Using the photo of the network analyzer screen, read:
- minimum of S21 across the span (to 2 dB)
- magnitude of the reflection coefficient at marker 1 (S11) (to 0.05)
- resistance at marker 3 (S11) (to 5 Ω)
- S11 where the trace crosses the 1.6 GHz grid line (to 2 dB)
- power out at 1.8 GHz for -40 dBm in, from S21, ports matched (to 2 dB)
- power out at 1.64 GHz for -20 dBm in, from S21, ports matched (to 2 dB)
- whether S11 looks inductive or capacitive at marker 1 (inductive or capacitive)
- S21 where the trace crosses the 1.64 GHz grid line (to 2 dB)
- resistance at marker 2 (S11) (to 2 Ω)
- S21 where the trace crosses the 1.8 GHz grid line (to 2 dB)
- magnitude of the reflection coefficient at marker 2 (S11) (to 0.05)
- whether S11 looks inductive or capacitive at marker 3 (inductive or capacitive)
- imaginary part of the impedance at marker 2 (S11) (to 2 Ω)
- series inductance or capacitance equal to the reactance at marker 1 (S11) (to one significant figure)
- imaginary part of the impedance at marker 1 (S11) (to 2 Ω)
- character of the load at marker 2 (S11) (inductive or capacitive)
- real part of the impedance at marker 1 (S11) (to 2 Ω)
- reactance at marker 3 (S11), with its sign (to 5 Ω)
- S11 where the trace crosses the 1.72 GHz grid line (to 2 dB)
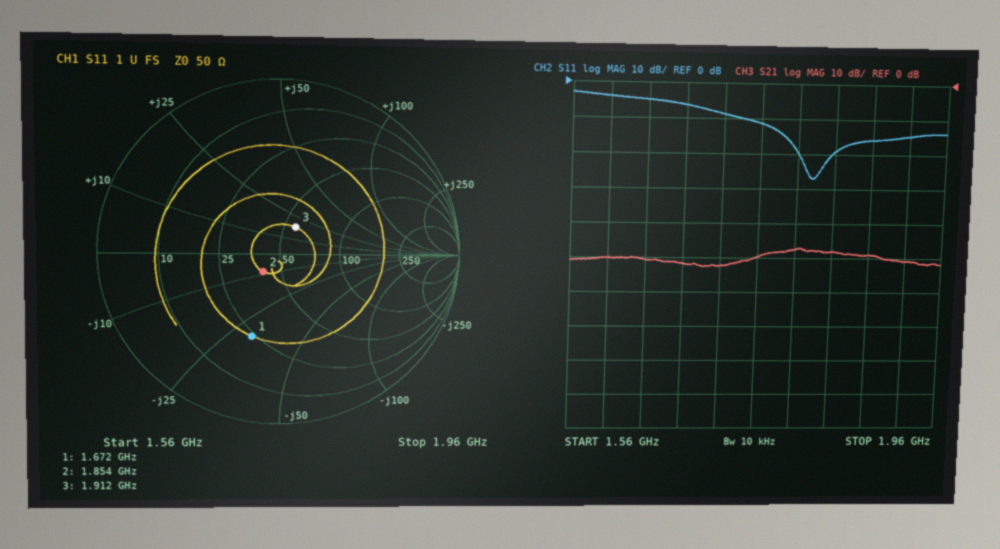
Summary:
-52 dB
0.50
55 Ω
-4 dB
-88 dBm
-70 dBm
capacitive
-50 dB
40 Ω
-48 dB
0.15
inductive
-8 Ω
3 pF
-30 Ω
capacitive
24 Ω
+20 Ω
-8 dB
